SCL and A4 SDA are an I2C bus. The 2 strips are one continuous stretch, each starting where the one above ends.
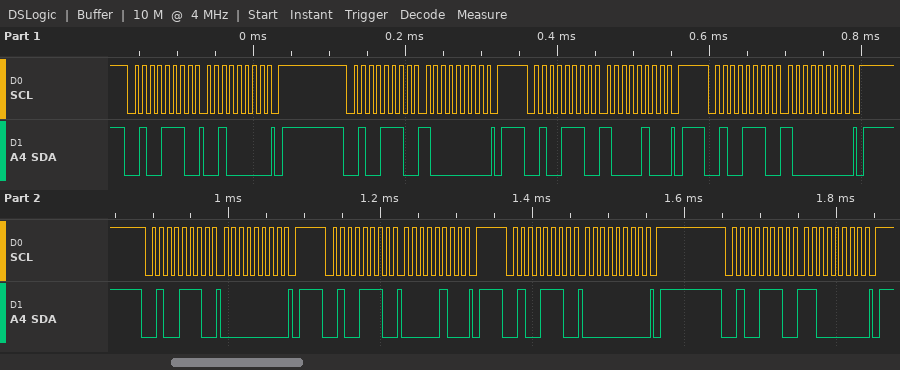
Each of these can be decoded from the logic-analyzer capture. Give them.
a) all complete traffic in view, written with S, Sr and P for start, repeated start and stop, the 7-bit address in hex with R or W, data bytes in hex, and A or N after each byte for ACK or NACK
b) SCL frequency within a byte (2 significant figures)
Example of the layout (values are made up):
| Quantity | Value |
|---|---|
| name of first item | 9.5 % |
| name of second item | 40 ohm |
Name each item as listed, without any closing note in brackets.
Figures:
| Quantity | Value |
|---|---|
| all complete traffic in view, written with S, Sr and P for start, repeated start and stop, the 7-bit address in hex with R or W, data bytes in hex, and A or N after each byte for ACK or NACK | S 27W A 20 A P S 27W A 80 A P S 27W A 84 A P S 27W A 80 A P S 27W A 00 A P S 27W A 04 A P S 27W A 00 A P S 27W A C0 A P |
| SCL frequency within a byte | 100 kHz |
